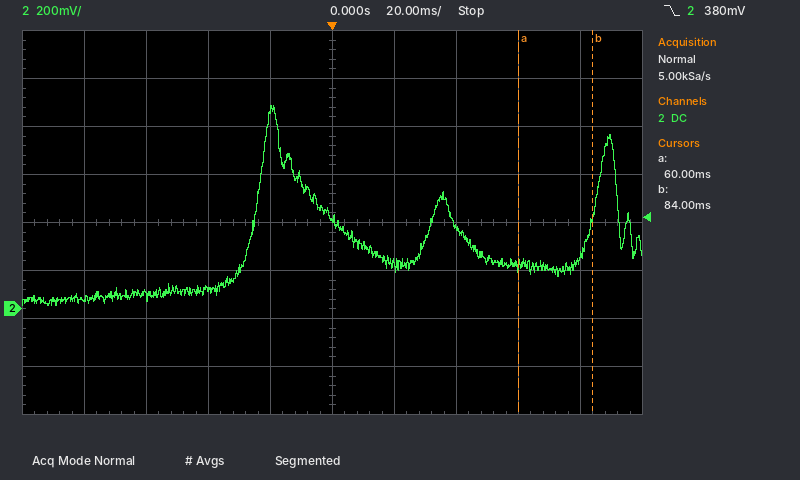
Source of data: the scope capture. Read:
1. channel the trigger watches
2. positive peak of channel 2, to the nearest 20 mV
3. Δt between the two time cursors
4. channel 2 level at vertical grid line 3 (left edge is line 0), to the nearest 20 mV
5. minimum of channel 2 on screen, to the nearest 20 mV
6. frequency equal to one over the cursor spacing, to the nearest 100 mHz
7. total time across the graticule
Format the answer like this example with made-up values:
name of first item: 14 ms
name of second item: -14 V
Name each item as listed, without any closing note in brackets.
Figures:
channel the trigger watches: channel 2
positive peak of channel 2, to the nearest 20 mV: 840 mV
Δt between the two time cursors: 24 ms
channel 2 level at vertical grid line 3 (left edge is line 0), to the nearest 20 mV: 80 mV
minimum of channel 2 on screen, to the nearest 20 mV: 20 mV
frequency equal to one over the cursor spacing, to the nearest 100 mHz: 41.7 Hz
total time across the graticule: 200 ms
